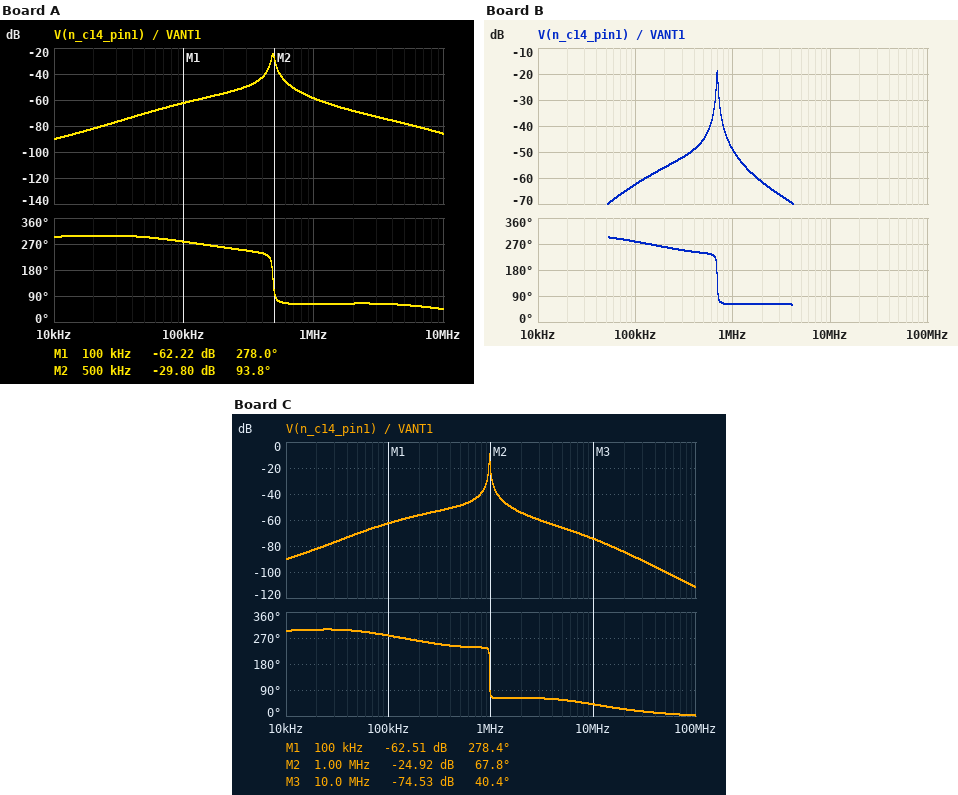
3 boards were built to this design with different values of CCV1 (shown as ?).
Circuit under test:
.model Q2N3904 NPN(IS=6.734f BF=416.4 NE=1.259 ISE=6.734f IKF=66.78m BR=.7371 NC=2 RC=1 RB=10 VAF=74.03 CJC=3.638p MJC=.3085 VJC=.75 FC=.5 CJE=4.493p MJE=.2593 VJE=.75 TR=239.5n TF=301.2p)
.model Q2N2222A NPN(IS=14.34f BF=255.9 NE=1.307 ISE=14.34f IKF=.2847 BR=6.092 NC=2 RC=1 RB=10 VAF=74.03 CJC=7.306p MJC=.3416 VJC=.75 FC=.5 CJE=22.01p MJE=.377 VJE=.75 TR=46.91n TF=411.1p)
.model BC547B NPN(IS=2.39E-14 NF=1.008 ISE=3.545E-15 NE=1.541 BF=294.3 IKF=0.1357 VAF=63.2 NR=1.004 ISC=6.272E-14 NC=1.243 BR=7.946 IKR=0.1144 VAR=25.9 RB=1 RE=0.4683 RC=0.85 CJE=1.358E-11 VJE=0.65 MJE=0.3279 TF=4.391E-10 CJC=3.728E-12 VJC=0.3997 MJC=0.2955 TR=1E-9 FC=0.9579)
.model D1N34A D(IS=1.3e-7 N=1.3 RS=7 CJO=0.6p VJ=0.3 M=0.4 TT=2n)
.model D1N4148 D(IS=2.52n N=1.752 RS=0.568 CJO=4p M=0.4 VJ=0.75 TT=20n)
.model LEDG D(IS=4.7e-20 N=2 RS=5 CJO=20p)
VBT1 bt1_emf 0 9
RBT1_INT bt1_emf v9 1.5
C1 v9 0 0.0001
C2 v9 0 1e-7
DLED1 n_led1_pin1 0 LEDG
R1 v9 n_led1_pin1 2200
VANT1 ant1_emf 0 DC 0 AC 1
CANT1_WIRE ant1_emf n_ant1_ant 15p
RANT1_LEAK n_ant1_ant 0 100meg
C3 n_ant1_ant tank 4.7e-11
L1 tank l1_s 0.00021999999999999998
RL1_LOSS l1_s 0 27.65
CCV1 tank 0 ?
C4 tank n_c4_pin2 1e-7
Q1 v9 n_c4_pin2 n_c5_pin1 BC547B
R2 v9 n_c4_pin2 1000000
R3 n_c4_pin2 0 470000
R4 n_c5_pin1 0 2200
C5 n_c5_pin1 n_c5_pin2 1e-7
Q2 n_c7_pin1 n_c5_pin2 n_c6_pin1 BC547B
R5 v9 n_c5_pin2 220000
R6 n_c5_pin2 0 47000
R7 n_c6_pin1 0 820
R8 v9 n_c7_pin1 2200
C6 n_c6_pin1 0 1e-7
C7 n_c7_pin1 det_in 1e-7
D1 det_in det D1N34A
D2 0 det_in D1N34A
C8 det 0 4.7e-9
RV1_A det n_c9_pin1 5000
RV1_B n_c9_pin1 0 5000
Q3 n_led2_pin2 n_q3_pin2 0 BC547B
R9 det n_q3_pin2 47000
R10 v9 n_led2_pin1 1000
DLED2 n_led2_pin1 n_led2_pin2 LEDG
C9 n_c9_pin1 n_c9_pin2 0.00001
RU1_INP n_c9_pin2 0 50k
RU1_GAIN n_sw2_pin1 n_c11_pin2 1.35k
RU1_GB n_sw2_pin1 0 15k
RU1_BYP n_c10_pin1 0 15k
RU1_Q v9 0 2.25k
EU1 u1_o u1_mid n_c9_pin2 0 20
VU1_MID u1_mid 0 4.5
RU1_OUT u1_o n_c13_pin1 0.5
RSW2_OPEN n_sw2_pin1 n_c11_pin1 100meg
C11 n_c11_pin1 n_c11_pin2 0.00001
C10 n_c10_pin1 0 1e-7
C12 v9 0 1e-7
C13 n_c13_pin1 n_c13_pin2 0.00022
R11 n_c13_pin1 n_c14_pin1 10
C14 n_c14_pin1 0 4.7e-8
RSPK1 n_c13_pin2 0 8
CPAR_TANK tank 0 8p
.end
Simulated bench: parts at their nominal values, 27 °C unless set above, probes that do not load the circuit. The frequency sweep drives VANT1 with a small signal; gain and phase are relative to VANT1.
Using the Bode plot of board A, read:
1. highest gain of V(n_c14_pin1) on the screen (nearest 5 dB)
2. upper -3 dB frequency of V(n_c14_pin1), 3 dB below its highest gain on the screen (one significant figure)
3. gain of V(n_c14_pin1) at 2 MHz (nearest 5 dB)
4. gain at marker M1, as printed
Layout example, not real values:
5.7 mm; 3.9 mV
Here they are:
-25 dB; 500 kHz; -70 dB; -62.22 dB
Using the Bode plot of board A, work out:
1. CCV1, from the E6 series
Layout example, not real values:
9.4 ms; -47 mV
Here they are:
470 pF
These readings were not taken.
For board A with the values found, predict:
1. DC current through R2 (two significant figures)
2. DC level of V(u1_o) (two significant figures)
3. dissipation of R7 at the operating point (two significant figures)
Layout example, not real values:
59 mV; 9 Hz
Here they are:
6.8 µA; 4.5 V; 820 µW
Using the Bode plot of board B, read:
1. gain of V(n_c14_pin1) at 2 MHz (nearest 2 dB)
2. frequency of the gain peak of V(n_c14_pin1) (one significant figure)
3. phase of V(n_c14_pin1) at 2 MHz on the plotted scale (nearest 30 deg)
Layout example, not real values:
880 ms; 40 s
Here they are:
-62 dB; 700 kHz; 60 deg
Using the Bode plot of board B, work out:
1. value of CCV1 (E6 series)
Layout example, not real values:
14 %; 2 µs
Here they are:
220 pF
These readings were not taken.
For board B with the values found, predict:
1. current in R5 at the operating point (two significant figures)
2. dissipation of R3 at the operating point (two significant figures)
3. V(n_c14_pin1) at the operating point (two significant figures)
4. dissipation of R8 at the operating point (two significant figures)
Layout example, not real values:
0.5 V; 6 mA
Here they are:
34 µA; 10 µW; 4.5 V; 2.2 mW
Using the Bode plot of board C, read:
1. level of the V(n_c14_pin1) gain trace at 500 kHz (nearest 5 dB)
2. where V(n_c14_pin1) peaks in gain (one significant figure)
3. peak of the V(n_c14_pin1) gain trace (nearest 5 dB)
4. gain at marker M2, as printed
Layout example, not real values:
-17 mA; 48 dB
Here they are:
-50 dB; 1 MHz; -10 dB; -24.92 dB
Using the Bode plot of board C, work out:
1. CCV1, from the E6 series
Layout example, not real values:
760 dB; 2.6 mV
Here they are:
100 pF
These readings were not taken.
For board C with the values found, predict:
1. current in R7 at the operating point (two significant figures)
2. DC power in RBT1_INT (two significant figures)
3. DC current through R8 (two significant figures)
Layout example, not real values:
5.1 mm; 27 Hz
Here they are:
1.0 mA; 120 µW; 1.0 mA
